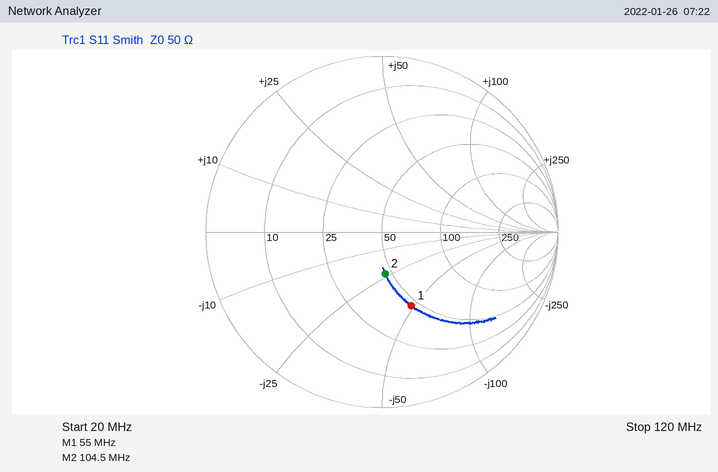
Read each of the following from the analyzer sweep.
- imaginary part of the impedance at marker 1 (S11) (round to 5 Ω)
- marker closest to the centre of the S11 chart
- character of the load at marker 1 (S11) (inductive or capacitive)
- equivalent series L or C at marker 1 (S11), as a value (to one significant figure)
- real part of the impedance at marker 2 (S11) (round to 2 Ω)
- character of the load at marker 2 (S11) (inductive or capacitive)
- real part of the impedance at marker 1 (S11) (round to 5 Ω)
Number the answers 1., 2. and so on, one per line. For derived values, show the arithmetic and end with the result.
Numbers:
1. -50 Ω
2. marker 2
3. capacitive
4. C = 1/(2π × 55 MHz × 50 Ω) ≈ 57.9 pF, so 60 pF to one significant figure
5. 46 Ω
6. capacitive
7. 45 Ω
